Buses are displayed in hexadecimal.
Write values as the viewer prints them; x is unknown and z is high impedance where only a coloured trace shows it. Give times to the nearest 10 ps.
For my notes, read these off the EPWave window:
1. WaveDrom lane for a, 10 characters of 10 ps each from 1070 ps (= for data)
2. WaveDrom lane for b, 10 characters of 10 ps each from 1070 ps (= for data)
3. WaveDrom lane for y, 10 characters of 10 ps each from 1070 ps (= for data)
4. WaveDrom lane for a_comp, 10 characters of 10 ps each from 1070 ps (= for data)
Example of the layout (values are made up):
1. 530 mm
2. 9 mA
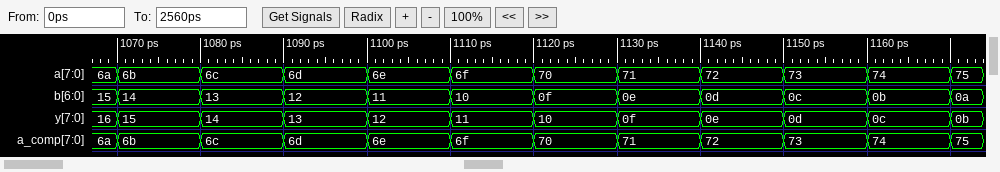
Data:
1. {name: 'a', wave: '==========', data: '6b 6c 6d 6e 6f 70 71 72 73 74'}
2. {name: 'b', wave: '==========', data: '14 13 12 11 10 0f 0e 0d 0c 0b'}
3. {name: 'y', wave: '==========', data: '15 14 13 12 11 10 0f 0e 0d 0c'}
4. {name: 'a_comp', wave: '==========', data: '6b 6c 6d 6e 6f 70 71 72 73 74'}
